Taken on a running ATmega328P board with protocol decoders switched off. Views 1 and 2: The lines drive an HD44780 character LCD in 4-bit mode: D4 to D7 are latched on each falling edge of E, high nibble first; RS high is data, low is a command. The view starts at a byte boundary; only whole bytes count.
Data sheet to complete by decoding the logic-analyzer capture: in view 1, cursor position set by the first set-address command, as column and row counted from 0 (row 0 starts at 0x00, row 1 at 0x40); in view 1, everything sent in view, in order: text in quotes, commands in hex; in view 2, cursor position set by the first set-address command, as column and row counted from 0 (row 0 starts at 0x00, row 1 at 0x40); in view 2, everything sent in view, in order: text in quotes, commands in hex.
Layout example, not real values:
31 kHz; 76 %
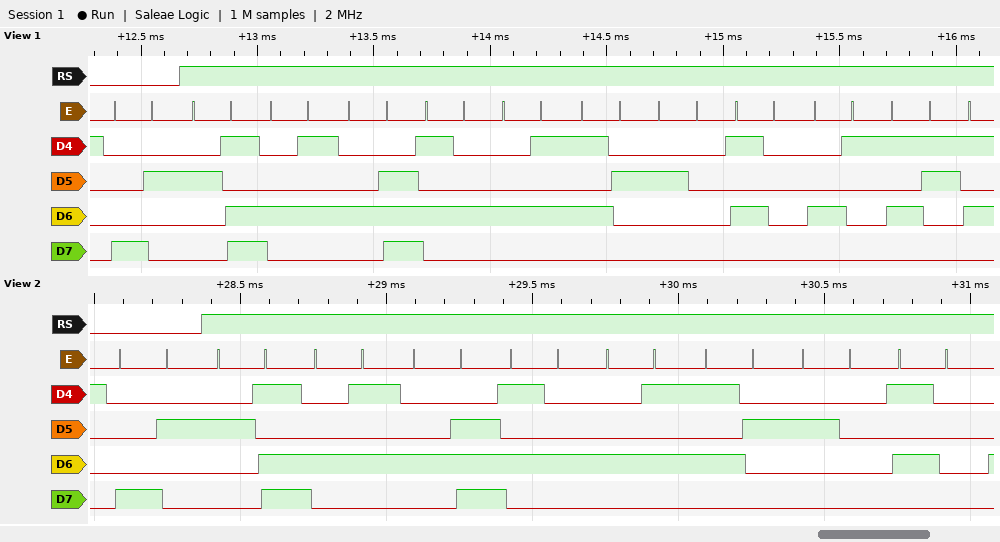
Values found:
column 2, row 0; 0x82 "-ENTER PAS"; column 2, row 0; 0x82 "-ENTER P"
